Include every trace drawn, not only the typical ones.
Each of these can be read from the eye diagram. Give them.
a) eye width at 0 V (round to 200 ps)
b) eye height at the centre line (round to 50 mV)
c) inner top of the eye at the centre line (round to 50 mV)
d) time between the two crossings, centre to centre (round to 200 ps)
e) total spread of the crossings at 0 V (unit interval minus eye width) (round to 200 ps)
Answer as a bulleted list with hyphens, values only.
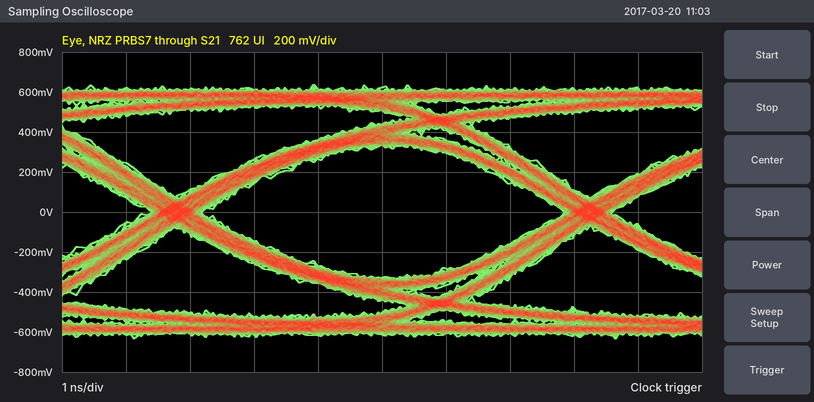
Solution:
- 5.6 ns
- 650 mV
- 350 mV
- 6.4 ns
- 800 ps
